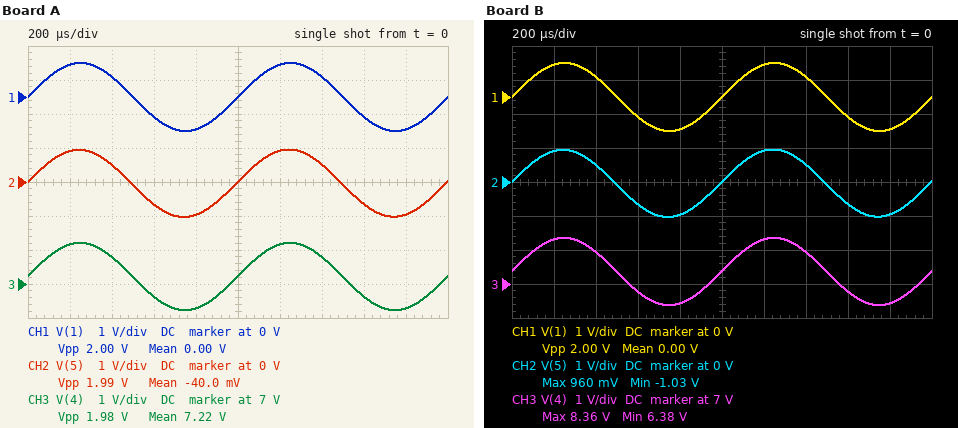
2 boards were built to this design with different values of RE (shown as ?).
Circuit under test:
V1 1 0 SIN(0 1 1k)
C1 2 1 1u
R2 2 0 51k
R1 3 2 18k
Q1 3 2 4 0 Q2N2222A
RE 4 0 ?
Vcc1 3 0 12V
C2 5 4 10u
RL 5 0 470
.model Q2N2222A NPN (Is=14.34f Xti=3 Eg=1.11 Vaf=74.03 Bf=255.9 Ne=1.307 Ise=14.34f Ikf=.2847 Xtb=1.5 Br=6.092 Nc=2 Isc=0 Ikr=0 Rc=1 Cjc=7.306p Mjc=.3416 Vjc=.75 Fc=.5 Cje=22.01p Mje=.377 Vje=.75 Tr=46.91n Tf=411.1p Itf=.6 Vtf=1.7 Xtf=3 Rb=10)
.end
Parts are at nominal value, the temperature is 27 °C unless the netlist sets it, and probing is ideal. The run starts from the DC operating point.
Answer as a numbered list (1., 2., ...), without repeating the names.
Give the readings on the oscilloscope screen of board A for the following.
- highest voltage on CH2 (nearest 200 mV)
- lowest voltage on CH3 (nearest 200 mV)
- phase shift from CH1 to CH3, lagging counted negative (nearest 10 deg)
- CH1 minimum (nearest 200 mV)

1. 1.0 V
2. 6.2 V
3. 0 deg
4. -1.0 V
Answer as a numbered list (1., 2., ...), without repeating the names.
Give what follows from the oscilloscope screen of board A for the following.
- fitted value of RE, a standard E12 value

1. 560 Ω
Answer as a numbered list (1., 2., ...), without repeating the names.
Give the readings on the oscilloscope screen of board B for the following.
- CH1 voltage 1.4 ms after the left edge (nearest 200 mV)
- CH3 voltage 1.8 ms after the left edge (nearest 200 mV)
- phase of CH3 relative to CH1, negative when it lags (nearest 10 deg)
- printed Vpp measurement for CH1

1. 600 mV
2. 6.4 V
3. 0 deg
4. 2.00 V
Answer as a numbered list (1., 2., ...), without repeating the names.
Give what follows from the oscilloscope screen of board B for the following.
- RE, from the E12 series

1. 680 Ω
